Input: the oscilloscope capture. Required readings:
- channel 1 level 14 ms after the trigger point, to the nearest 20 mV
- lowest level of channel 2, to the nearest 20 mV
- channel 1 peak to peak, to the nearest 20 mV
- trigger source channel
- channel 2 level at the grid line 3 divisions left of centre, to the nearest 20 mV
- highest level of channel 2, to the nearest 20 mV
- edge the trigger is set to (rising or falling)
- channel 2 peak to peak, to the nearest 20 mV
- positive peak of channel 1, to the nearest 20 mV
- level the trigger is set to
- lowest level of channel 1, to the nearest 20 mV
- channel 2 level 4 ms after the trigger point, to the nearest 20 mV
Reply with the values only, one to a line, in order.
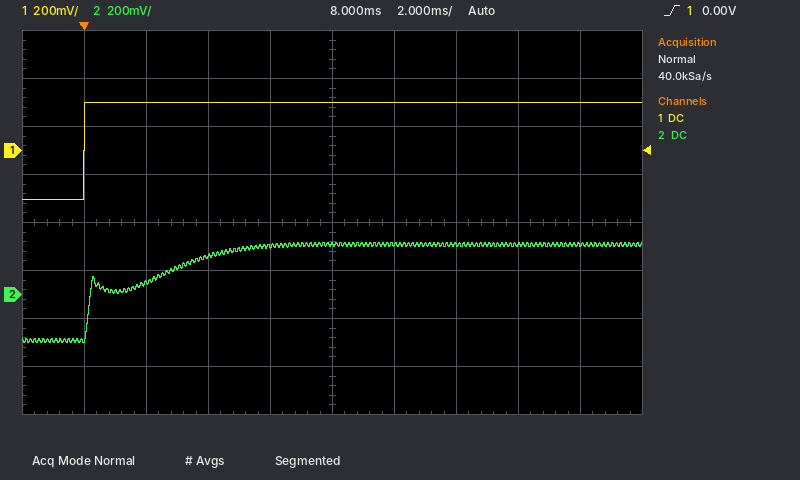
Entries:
200 mV
-200 mV
400 mV
channel 1
40 mV
220 mV
rising
420 mV
200 mV
0.00 V
-200 mV
160 mV
